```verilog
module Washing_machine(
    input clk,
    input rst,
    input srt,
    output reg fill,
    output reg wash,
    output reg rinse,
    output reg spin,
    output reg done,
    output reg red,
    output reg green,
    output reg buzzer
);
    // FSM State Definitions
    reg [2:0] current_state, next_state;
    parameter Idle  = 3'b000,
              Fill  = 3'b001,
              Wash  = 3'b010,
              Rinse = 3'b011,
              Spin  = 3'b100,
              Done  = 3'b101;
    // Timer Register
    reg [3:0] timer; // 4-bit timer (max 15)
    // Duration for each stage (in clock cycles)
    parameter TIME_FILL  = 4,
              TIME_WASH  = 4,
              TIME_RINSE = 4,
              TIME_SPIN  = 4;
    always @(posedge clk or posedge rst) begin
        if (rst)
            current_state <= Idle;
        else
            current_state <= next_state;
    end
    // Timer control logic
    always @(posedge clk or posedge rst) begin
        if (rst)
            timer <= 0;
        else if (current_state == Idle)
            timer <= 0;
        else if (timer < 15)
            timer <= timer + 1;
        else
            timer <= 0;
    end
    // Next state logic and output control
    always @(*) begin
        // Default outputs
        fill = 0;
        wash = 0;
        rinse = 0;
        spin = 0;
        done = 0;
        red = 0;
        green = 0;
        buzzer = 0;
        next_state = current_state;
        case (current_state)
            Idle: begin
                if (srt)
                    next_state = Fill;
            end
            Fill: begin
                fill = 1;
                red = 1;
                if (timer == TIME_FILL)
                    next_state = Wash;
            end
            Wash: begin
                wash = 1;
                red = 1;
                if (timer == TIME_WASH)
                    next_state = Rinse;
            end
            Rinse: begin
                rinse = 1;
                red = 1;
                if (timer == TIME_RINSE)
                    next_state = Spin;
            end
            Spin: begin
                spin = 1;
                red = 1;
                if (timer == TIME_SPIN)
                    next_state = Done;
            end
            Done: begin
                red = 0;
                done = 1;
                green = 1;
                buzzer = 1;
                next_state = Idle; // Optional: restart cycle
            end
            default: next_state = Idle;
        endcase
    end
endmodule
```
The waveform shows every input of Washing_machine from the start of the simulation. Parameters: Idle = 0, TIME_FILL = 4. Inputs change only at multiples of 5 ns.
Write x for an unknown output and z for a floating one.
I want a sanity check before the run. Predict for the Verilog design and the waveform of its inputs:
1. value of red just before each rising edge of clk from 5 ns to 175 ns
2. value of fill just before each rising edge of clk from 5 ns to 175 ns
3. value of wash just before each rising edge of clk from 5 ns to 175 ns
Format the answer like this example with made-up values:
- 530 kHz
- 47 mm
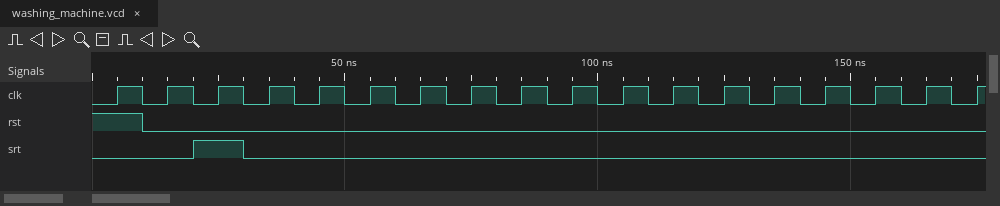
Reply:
- 0 0 0 1 1 1 1 1 1 1 1 1 1 1 1 1 1 1
- 0 0 0 1 1 1 1 1 0 0 0 0 0 0 0 0 0 0
- 0 0 0 0 0 0 0 0 1 1 1 1 1 1 1 1 1 1
